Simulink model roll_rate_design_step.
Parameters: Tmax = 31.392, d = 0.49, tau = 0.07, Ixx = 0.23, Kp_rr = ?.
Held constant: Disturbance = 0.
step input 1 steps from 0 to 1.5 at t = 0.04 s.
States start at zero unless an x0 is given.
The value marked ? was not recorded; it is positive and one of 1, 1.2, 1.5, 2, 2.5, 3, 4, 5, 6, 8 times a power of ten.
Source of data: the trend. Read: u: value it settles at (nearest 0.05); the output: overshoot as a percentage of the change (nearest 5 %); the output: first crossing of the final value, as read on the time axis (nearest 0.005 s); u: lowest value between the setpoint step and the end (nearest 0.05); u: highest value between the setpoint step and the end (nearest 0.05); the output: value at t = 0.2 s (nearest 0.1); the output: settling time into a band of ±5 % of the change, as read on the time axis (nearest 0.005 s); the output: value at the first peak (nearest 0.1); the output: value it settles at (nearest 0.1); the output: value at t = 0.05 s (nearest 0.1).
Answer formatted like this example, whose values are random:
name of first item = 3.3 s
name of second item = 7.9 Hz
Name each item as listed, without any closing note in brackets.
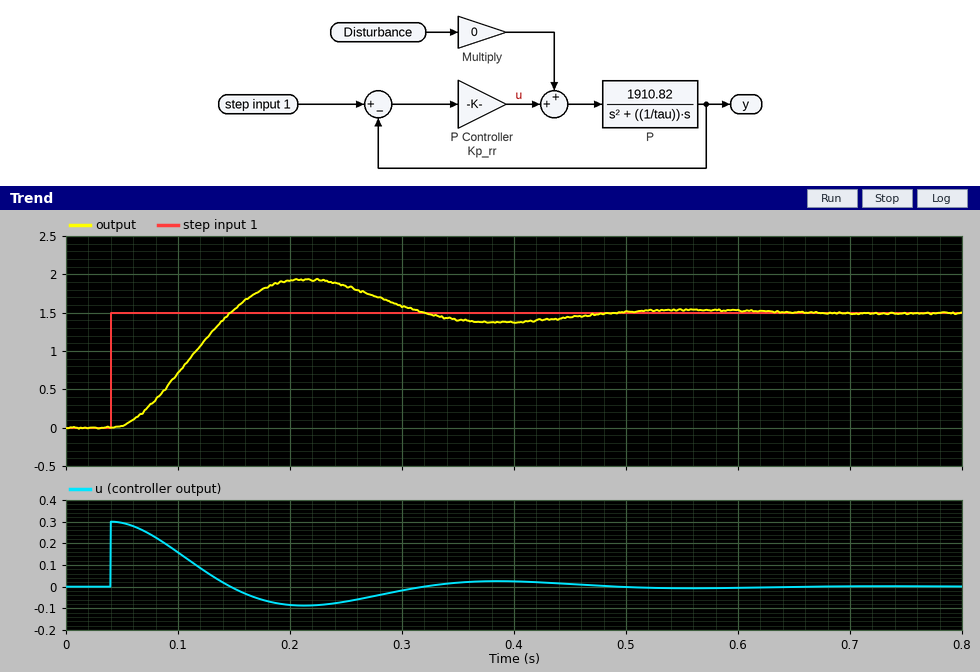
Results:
u: value it settles at = 0.00
the output: overshoot as a percentage of the change = 30 %
the output: first crossing of the final value, as read on the time axis = 0.145 s
u: lowest value between the setpoint step and the end = -0.10
u: highest value between the setpoint step and the end = 0.30
the output: value at t = 0.2 s = 1.9
the output: settling time into a band of ±5 % of the change, as read on the time axis = 0.440 s
the output: value at the first peak = 1.9
the output: value it settles at = 1.5
the output: value at t = 0.05 s = 0.0
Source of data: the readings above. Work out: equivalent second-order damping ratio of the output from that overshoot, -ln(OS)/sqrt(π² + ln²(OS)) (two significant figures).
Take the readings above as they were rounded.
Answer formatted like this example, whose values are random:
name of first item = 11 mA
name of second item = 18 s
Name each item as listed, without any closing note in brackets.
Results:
equivalent second-order damping ratio of the output from that overshoot, -ln(OS)/sqrt(π² + ln²(OS)) = 0.36
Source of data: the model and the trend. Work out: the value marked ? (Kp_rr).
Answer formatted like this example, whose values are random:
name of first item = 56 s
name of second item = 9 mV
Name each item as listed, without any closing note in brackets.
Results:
the value marked ? = 0.2
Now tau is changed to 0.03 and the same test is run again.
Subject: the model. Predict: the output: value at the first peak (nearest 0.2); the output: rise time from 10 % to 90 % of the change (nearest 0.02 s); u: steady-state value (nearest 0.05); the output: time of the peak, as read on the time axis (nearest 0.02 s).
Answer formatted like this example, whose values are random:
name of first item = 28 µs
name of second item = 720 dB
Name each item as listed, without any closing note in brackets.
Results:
the output: value at the first peak = 1.6
the output: rise time from 10 % to 90 % of the change = 0.06 s
u: steady-state value = 0.00
the output: time of the peak, as read on the time axis = 0.16 s
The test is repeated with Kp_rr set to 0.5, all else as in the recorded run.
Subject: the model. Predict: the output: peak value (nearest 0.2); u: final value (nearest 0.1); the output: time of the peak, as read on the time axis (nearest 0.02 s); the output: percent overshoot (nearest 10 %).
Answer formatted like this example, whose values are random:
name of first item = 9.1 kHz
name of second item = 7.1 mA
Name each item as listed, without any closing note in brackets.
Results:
the output: peak value = 2.2
u: final value = 0.0
the output: time of the peak, as read on the time axis = 0.14 s
the output: percent overshoot = 50 %
